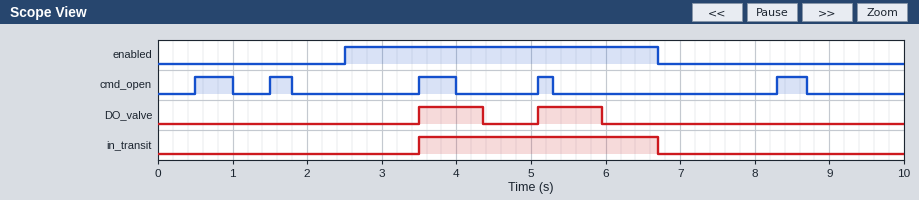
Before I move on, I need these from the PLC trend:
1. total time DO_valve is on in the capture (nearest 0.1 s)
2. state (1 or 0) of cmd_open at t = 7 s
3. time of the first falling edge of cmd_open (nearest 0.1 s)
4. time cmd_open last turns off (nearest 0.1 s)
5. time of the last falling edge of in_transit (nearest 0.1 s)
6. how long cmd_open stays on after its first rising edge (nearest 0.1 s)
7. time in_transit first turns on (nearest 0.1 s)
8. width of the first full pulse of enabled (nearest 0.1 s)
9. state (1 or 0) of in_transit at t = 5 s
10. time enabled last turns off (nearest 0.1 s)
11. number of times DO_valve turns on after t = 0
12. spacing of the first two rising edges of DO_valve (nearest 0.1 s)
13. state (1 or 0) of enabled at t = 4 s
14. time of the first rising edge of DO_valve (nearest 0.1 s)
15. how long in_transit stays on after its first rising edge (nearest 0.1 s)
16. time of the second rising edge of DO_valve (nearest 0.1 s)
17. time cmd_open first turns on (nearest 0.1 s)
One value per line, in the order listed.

1.7 s
0
1.0 s
8.7 s
6.7 s
0.5 s
3.5 s
4.2 s
1
6.7 s
2
1.6 s
1
3.5 s
3.2 s
5.1 s
0.5 s
